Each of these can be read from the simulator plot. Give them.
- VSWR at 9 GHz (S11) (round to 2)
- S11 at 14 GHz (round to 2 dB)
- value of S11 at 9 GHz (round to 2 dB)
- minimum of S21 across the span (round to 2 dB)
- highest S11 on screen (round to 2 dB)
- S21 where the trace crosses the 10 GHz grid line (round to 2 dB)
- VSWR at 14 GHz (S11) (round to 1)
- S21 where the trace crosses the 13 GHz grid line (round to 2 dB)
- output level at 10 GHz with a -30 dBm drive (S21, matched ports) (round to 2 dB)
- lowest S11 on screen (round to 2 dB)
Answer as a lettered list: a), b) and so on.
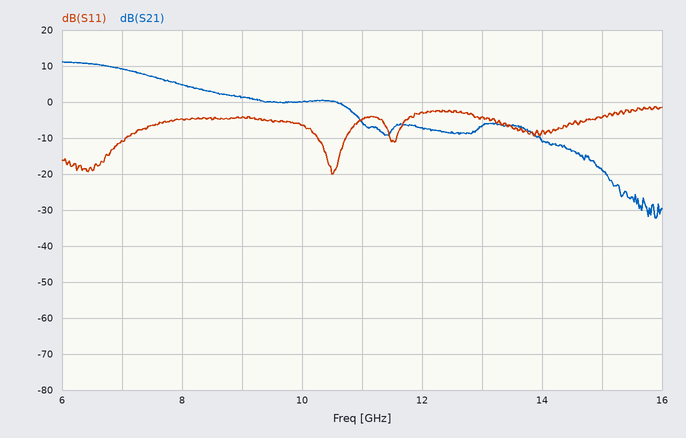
a) 4
b) -8 dB
c) -4 dB
d) -32 dB
e) -2 dB
f) 0 dB
g) 2
h) -6 dB
i) -30 dBm
j) -20 dB
